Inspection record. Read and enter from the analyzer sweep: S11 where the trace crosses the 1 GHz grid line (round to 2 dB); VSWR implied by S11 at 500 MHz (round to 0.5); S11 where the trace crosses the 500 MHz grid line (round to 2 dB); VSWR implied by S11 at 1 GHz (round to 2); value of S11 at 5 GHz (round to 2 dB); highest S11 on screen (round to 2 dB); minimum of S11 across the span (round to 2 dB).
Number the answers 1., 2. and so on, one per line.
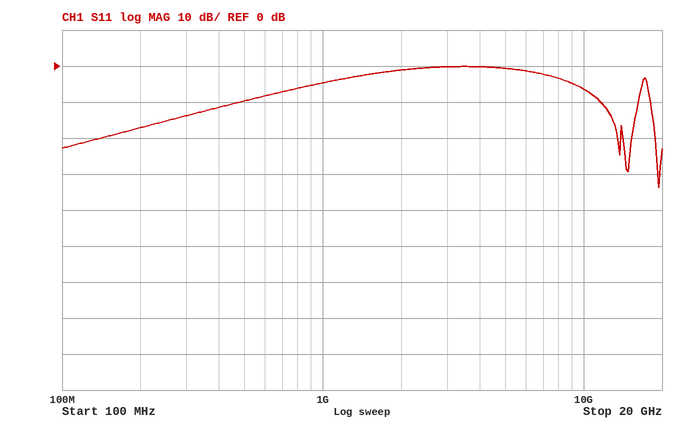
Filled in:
1. -4 dB
2. 2.0
3. -10 dB
4. 4
5. 0 dB
6. 0 dB
7. -34 dB
